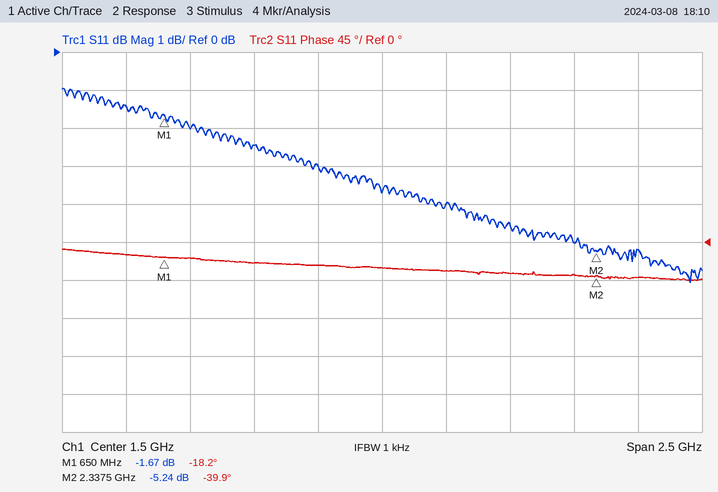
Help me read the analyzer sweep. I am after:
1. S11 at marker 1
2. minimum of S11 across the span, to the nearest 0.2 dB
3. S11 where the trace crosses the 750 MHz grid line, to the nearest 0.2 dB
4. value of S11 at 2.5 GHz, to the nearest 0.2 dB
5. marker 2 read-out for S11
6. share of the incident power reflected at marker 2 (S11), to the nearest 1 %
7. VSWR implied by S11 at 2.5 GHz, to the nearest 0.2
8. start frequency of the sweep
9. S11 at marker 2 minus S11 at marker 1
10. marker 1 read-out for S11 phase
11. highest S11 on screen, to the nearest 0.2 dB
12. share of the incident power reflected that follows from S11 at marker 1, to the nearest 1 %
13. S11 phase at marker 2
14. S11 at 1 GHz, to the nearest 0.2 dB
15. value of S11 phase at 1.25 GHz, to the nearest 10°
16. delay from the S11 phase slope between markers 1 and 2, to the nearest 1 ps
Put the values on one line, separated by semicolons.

-1.67 dB; -6.0 dB; -2.0 dB; -5.2 dB; -5.24 dB; 30 %; 3.4; 250 MHz; -3.57 dB; -18.2°; -1.0 dB; 68 %; -39.9°; -2.4 dB; -30°; 36 ps
